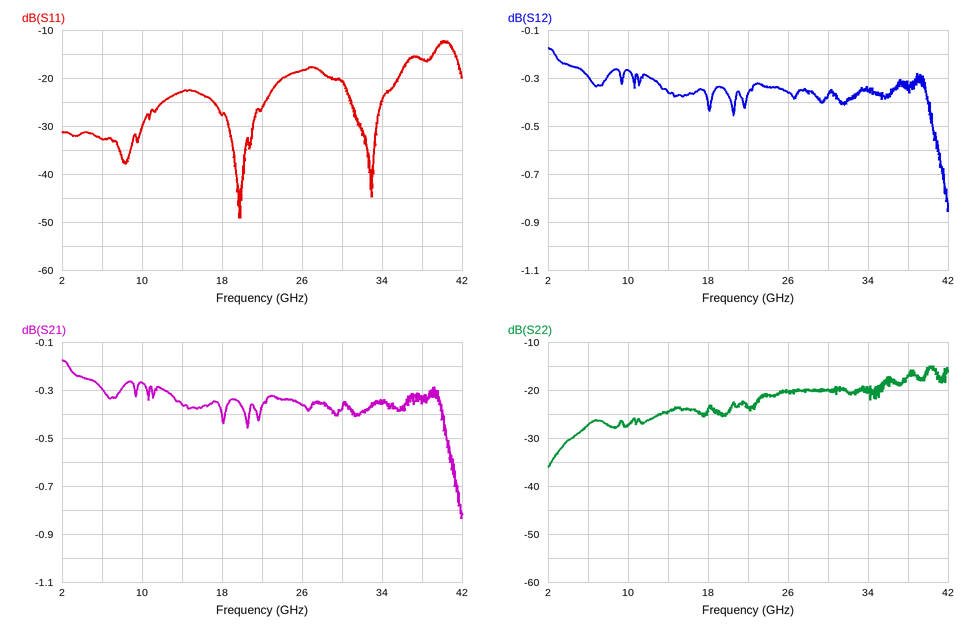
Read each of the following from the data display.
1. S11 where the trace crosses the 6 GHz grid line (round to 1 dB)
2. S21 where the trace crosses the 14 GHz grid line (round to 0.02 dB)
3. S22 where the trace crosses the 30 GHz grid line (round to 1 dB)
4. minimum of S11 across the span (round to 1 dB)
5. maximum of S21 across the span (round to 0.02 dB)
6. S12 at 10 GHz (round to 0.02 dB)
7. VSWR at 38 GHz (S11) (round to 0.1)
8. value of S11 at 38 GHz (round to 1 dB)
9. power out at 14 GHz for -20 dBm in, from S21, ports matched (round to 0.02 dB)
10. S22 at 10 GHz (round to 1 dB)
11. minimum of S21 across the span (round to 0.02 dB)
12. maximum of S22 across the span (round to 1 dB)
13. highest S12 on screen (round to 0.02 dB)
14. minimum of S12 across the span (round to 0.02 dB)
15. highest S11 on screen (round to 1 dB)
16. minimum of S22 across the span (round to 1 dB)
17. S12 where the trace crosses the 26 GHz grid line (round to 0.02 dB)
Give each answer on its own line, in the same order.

-33 dB
-0.36 dB
-20 dB
-49 dB
-0.18 dB
-0.26 dB
1.4
-16 dB
-20.36 dBm
-27 dB
-0.84 dB
-15 dB
-0.18 dB
-0.86 dB
-12 dB
-36 dB
-0.36 dB
